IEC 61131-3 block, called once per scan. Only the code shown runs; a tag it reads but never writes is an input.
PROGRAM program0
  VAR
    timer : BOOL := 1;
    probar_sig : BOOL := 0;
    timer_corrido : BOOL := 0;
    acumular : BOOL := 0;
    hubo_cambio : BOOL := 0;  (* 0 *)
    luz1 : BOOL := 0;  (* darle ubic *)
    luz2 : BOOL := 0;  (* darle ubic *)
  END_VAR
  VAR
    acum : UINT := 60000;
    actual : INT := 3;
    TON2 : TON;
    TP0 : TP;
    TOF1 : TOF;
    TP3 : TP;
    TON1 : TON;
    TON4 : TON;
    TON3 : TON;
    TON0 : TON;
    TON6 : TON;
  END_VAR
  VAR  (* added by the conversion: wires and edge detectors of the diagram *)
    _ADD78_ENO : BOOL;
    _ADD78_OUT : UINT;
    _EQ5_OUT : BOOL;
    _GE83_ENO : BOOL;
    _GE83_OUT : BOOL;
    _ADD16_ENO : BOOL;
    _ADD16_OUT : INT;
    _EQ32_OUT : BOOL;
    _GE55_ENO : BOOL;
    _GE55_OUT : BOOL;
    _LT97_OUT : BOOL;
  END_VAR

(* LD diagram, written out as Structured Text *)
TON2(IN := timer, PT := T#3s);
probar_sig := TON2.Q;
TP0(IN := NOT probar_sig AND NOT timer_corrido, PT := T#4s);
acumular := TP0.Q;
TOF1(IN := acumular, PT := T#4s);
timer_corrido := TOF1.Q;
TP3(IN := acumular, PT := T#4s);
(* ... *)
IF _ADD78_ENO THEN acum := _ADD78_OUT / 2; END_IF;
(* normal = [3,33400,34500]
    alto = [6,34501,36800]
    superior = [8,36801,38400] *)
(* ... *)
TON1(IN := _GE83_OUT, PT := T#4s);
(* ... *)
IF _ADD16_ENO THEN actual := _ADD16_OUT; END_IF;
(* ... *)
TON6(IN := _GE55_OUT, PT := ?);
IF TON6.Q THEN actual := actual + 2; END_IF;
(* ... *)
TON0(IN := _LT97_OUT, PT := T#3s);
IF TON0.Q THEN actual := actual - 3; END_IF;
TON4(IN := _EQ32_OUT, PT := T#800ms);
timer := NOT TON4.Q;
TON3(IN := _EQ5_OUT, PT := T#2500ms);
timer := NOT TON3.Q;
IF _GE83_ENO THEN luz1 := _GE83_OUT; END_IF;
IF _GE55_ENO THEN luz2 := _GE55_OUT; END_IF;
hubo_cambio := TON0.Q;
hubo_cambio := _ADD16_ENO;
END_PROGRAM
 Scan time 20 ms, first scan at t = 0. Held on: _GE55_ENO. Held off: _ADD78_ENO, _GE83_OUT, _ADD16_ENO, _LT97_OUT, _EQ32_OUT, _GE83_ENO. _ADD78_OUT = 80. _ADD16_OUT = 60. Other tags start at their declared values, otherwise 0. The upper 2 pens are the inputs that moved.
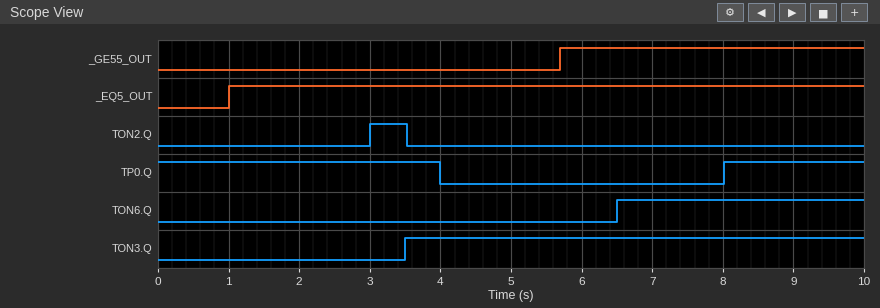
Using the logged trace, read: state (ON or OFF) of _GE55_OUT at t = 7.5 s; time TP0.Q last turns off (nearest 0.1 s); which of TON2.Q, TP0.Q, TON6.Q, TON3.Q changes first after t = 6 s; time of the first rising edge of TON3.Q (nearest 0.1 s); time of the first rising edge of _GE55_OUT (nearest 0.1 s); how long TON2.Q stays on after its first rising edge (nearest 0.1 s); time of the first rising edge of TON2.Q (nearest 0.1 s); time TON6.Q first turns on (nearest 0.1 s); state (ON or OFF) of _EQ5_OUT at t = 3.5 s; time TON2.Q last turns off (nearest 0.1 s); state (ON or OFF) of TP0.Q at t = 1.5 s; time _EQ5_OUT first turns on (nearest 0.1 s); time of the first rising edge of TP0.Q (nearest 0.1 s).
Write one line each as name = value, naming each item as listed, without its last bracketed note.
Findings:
state (ON or OFF) of _GE55_OUT at t = 7.5 s = ON
time TP0.Q last turns off = 4.0 s
which of TON2.Q, TP0.Q, TON6.Q, TON3.Q changes first after t = 6 s = TON6.Q
time of the first rising edge of TON3.Q = 3.5 s
time of the first rising edge of _GE55_OUT = 5.7 s
how long TON2.Q stays on after its first rising edge = 0.5 s
time of the first rising edge of TON2.Q = 3.0 s
time TON6.Q first turns on = 6.5 s
state (ON or OFF) of _EQ5_OUT at t = 3.5 s = ON
time TON2.Q last turns off = 3.5 s
state (ON or OFF) of TP0.Q at t = 1.5 s = ON
time _EQ5_OUT first turns on = 1.0 s
time of the first rising edge of TP0.Q = 8.0 s
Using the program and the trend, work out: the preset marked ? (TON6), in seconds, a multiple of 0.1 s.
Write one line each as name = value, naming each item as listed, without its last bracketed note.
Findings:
the preset marked ? (TON6), in seconds, a multiple of 0.1 s = 0.8 s
